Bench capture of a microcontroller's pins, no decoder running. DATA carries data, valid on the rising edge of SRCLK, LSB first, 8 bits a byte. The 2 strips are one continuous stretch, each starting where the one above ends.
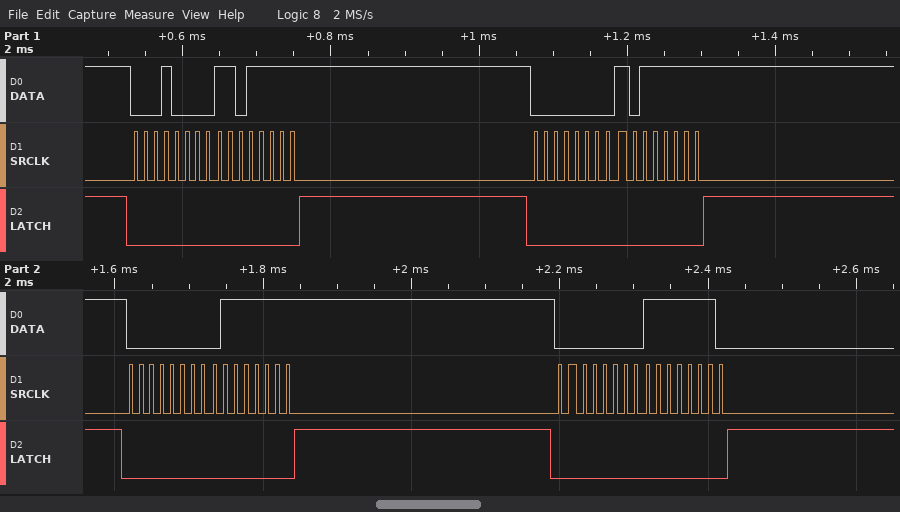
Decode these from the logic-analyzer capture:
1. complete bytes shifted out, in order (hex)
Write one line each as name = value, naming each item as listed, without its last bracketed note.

complete bytes shifted out, in order = 08 FB 00 FD 00 FE 00 7F
